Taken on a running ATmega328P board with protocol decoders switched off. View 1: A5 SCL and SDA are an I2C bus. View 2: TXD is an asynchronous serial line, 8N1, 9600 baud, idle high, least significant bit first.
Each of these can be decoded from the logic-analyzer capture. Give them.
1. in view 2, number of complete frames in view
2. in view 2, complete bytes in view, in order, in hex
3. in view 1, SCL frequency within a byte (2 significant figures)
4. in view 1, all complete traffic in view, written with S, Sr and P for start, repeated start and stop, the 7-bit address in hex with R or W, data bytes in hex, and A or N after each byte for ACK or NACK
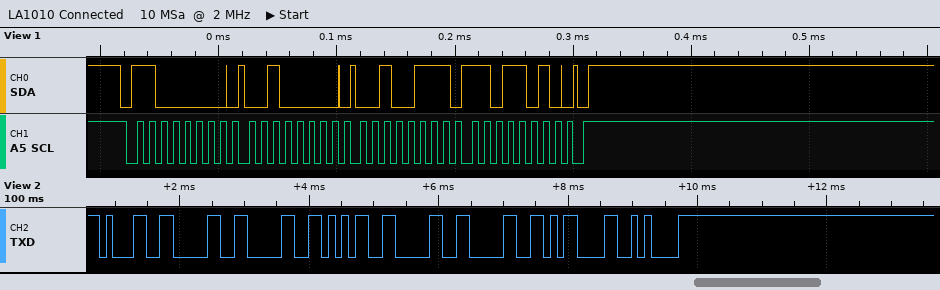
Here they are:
8
31 30 30 35 30 30 0D 0A
100 kHz
S 60W A 20 A 27 A DA A P
